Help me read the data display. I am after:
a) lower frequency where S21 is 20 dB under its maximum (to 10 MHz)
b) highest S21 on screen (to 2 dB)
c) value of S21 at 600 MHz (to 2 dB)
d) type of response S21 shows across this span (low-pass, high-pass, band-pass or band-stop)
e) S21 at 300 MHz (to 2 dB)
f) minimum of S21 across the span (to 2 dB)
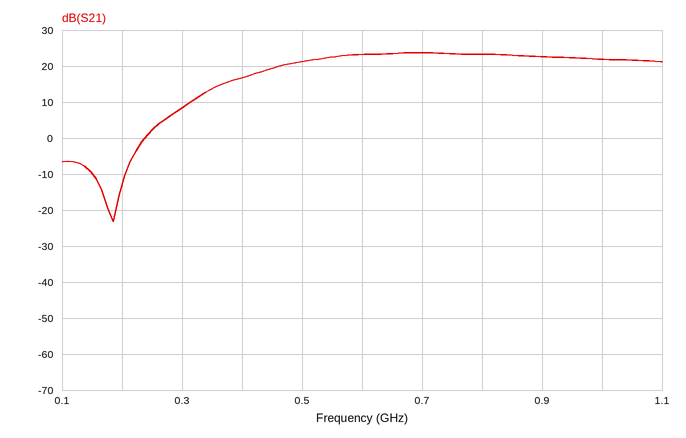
260 MHz
24 dB
24 dB
high-pass
8 dB
-24 dB
